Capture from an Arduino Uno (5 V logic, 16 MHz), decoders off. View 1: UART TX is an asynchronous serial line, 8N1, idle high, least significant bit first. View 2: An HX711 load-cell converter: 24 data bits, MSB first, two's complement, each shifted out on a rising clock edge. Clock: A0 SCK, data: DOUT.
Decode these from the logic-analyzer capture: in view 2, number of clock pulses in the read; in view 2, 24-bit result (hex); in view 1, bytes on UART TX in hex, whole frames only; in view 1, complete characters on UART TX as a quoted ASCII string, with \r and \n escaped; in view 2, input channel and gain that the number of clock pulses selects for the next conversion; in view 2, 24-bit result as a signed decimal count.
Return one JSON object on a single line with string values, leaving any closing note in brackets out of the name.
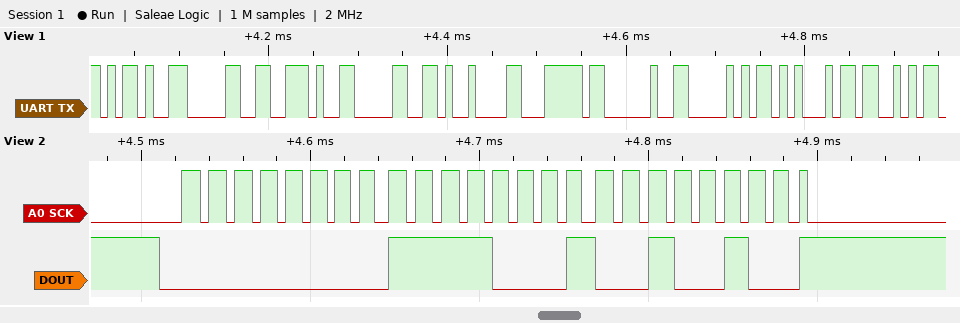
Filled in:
{"in view 2, number of clock pulses in the read": "25", "in view 2, 24-bit result": "0x00F124", "in view 1, bytes on UART TX in hex, whole frames only": "2D 30 2E 30 09 7C 20 50 45 53", "in view 1, complete characters on UART TX as a quoted ASCII string, with \\r and \\n escaped": "\"-0.0\\t| PES\"", "in view 2, input channel and gain that the number of clock pulses selects for the next conversion": "channel A, gain 128", "in view 2, 24-bit result as a signed decimal count": "61732"}
